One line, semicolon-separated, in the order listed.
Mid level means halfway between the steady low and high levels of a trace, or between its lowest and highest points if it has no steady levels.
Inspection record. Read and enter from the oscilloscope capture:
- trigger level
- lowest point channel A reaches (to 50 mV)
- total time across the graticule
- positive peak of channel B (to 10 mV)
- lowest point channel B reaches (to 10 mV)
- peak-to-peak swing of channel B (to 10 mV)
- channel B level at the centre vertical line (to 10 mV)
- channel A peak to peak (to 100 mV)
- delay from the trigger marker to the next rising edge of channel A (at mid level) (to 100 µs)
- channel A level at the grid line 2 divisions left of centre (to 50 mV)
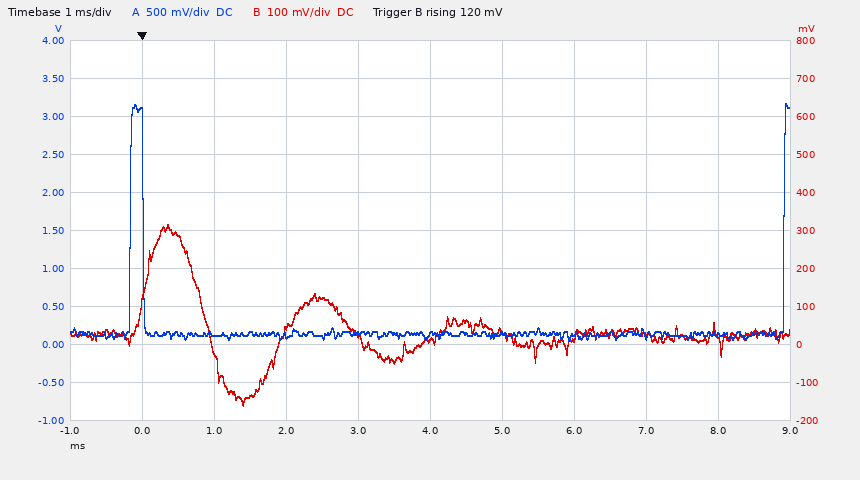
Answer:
120 mV; 50 mV; 10 ms; 320 mV; -160 mV; 480 mV; 10 mV; 3.10 V; 8.9 ms; 100 mV
